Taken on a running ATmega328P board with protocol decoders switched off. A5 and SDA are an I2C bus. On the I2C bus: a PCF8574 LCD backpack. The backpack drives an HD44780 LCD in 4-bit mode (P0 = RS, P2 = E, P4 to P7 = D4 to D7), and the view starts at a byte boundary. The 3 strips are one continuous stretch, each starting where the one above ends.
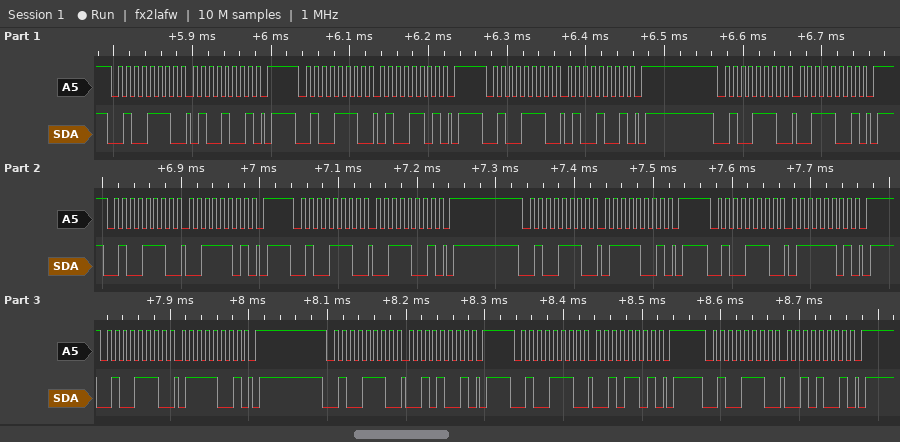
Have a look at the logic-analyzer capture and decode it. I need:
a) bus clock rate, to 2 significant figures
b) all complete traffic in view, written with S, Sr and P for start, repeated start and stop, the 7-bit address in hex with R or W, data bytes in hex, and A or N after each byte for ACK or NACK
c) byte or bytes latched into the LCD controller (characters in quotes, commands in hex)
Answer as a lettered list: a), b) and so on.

a) 100 kHz
b) S 27W A 49 A P S 27W A 4D A P S 27W A 49 A P S 27W A 39 A P S 27W A 3D A P S 27W A 39 A P S 27W A 79 A P S 27W A 7D A P S 27W A 79 A P S 27W A 29 A P S 27W A 2D A P S 27W A 29 A P
c) 'C' 'r'
